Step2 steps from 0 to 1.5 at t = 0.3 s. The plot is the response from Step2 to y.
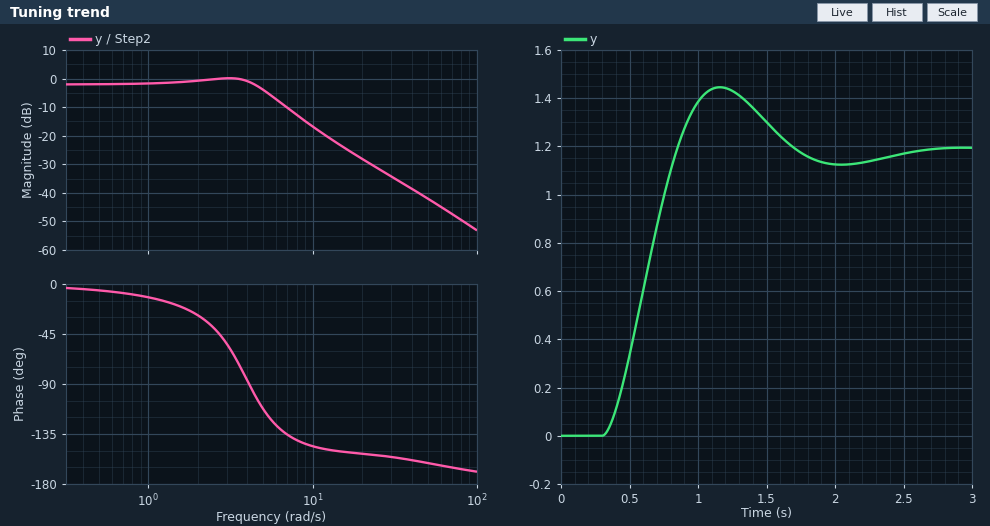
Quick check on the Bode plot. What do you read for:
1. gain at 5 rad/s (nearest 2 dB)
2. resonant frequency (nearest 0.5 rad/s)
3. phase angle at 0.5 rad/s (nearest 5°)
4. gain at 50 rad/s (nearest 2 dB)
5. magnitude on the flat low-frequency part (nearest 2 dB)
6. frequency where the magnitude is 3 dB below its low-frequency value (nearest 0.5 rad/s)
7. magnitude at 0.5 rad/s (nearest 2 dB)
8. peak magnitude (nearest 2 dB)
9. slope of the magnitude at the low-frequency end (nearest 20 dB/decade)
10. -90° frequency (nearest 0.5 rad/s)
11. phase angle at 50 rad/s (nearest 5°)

-4 dB
3.0 rad/s
-5°
-42 dB
-2 dB
5.5 rad/s
-2 dB
0 dB
0 dB/decade
4.0 rad/s
-160°
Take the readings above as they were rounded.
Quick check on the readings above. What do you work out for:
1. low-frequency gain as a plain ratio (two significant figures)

0.79
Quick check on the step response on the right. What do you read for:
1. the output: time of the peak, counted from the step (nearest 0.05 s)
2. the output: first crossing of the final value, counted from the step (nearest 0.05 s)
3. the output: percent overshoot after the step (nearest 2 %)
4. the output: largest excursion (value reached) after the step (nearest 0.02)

0.85 s
0.55 s
22 %
1.44
